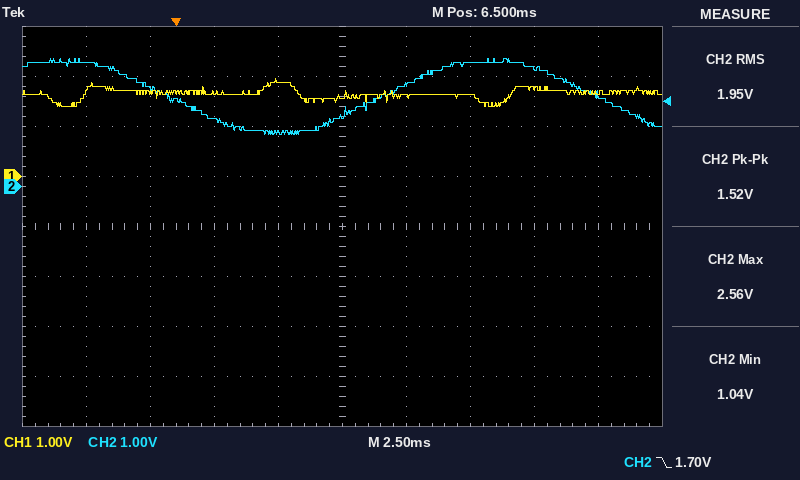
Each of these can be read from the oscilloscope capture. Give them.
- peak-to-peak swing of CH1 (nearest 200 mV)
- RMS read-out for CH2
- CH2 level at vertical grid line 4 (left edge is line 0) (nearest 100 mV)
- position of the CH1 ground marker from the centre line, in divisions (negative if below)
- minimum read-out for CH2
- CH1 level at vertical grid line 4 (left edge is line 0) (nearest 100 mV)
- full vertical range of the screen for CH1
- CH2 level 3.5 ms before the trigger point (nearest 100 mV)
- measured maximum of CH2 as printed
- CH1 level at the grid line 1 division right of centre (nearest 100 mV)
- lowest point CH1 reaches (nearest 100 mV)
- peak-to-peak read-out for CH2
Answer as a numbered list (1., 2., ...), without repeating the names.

1. 600 mV
2. 1.95 V
3. 1.1 V
4. +1.0 div
5. 1.04 V
6. 1.9 V
7. 8 V
8. 2.5 V
9. 2.56 V
10. 1.6 V
11. 1.4 V
12. 1.52 V
